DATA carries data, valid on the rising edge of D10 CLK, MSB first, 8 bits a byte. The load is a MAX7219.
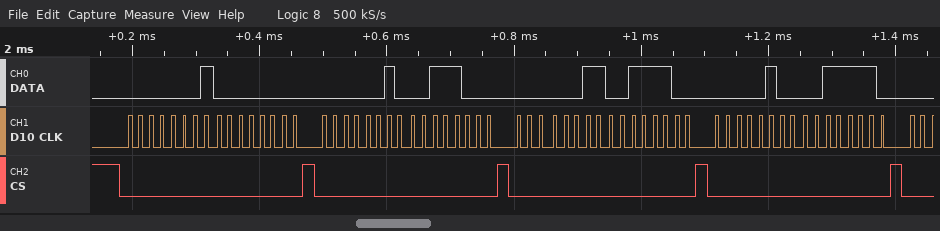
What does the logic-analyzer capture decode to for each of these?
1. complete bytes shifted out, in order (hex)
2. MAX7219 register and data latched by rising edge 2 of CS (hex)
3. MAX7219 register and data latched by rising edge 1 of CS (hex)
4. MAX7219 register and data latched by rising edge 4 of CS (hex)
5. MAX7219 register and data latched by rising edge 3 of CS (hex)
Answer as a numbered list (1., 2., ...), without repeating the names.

1. 01 00 02 38 03 3C 04 3E
2. register 0x2, data 0x38
3. register 0x1, data 0x00
4. register 0x4, data 0x3E
5. register 0x3, data 0x3C
